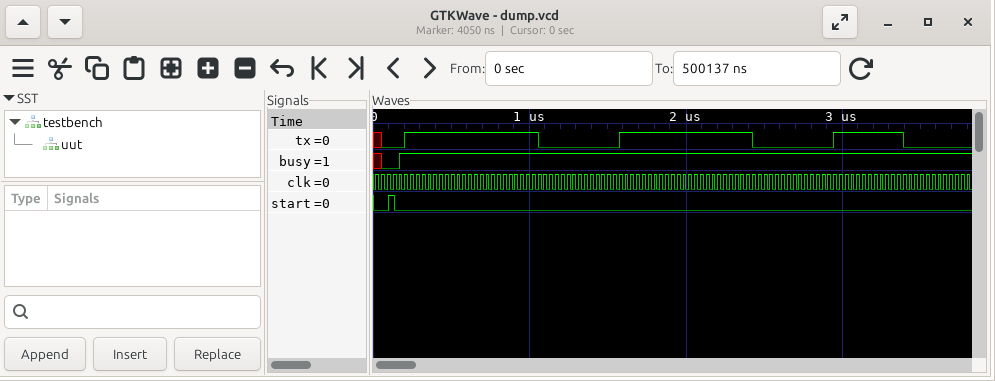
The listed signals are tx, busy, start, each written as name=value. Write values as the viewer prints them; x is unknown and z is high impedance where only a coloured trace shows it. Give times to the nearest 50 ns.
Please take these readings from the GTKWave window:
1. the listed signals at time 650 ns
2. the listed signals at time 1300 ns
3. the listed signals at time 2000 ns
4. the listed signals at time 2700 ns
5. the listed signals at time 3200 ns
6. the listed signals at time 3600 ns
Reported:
tx=1, busy=1, start=0
tx=0, busy=1, start=0
tx=1, busy=1, start=0
tx=0, busy=1, start=0
tx=1, busy=1, start=0
tx=0, busy=1, start=0
